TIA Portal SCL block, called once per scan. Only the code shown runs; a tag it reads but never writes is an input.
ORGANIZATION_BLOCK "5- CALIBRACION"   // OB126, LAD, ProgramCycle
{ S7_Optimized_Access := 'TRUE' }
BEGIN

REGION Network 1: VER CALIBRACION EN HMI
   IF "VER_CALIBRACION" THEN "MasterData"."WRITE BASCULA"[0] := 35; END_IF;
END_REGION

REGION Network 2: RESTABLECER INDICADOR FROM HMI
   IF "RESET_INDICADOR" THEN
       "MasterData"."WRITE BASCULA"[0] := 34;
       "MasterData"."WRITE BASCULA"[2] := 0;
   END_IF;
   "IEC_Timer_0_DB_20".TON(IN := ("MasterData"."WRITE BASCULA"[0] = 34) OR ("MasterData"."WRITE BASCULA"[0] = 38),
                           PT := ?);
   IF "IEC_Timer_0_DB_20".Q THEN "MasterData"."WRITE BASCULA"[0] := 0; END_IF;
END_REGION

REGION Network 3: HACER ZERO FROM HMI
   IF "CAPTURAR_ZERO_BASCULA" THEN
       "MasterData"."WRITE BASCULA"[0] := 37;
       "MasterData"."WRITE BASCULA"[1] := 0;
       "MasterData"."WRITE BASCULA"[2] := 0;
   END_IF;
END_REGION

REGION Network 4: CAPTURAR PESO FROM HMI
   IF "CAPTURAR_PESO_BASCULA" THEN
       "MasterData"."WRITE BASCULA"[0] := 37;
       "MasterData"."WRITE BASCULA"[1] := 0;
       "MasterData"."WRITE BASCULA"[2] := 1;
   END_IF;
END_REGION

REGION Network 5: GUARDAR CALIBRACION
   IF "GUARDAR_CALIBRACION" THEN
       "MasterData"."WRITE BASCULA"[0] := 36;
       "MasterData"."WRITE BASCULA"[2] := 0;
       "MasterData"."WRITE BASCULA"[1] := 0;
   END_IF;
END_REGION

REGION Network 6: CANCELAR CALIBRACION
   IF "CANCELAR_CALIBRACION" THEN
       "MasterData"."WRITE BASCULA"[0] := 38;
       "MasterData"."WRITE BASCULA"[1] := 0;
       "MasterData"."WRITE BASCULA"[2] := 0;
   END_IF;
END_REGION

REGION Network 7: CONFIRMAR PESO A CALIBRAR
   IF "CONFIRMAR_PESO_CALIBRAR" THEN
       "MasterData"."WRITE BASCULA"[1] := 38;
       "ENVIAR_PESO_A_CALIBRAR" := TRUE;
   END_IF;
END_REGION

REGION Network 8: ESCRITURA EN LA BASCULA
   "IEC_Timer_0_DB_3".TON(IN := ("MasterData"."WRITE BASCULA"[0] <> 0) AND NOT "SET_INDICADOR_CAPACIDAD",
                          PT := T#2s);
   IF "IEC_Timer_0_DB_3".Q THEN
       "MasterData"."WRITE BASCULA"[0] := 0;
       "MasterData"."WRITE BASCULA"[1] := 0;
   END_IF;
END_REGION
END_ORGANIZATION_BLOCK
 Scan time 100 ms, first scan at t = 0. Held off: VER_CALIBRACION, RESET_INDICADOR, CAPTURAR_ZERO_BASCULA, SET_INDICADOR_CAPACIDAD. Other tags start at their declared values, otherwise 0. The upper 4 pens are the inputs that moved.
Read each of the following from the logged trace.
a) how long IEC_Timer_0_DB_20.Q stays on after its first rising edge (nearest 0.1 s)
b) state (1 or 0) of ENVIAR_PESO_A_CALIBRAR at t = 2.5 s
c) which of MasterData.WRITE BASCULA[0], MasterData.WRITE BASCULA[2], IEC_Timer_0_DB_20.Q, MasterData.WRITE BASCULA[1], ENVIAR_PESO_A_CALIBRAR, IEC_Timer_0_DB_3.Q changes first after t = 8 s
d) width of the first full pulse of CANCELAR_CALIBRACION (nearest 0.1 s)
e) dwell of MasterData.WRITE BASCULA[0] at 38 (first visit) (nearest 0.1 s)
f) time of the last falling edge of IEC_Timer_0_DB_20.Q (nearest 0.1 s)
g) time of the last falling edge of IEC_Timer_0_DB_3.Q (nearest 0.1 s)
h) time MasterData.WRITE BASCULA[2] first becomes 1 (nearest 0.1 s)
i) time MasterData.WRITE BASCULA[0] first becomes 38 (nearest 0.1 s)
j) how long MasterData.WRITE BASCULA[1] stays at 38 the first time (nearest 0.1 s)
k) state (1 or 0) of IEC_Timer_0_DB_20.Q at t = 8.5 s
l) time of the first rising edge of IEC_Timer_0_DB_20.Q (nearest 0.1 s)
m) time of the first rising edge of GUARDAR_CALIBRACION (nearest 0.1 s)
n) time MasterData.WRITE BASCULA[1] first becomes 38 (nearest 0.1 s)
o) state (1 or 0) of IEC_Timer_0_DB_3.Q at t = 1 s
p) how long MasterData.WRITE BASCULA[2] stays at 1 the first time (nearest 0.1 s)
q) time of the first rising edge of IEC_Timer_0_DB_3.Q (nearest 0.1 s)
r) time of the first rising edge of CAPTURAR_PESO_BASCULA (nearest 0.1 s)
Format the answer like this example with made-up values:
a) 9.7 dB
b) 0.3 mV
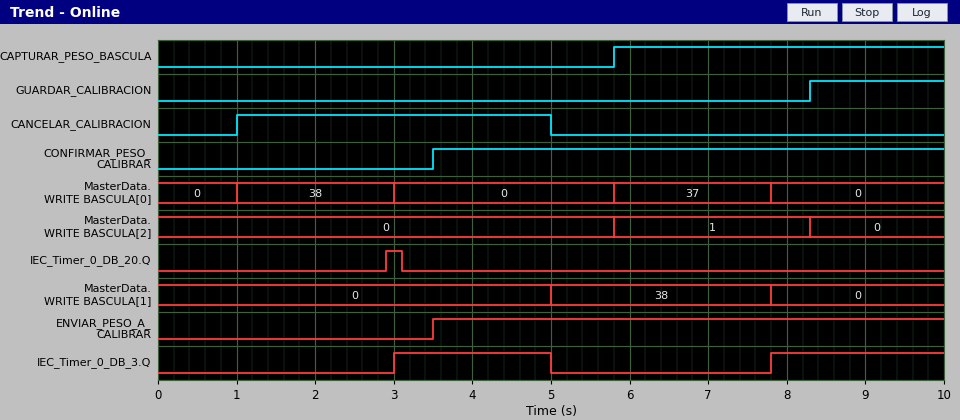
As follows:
a) 0.2 s
b) 0
c) MasterData.WRITE BASCULA[2]
d) 4.0 s
e) 2.0 s
f) 3.1 s
g) 5.0 s
h) 5.8 s
i) 1.0 s
j) 2.8 s
k) 0
l) 2.9 s
m) 8.3 s
n) 5.0 s
o) 0
p) 2.5 s
q) 3.0 s
r) 5.8 s
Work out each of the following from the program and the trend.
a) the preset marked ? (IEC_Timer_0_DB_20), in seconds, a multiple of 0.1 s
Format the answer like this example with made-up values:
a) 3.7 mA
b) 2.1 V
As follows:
a) 1.8 s
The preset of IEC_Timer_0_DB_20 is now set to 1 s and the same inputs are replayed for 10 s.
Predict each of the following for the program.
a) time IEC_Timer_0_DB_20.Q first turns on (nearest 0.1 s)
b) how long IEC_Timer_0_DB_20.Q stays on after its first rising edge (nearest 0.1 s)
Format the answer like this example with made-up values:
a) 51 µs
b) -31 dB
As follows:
a) 2.1 s
b) 1.0 s
